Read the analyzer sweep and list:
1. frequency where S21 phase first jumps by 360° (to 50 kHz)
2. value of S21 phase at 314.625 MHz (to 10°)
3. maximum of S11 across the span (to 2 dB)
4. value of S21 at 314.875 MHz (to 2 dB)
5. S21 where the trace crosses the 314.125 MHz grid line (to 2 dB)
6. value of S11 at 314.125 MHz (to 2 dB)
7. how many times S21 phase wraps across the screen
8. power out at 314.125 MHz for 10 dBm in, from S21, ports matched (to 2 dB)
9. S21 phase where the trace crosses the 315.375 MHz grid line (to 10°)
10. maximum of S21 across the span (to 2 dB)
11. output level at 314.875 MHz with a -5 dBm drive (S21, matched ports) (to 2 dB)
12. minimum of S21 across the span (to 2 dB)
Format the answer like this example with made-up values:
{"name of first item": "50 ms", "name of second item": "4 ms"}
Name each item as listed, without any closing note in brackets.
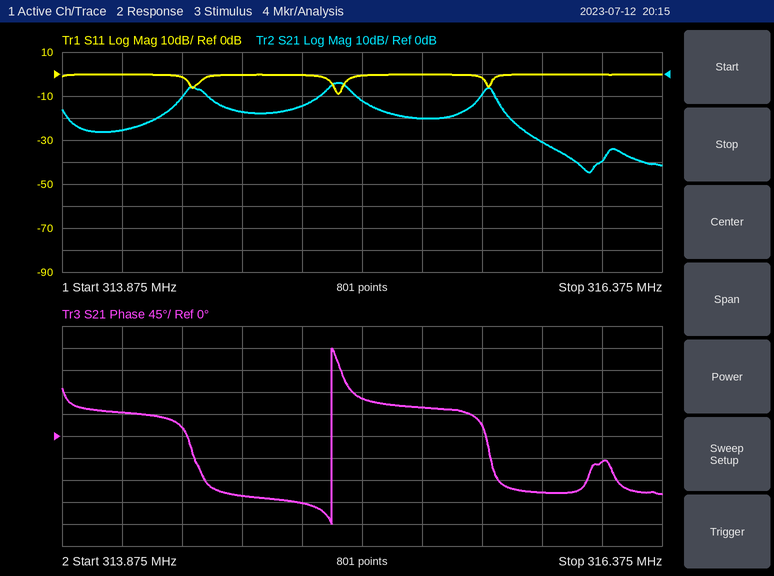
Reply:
{"frequency where S21 phase first jumps by 360°": "315.00 MHz", "value of S21 phase at 314.625 MHz": "-120°", "maximum of S11 across the span": "0 dB", "value of S21 at 314.875 MHz": "-14 dB", "S21 where the trace crosses the 314.125 MHz grid line": "-26 dB", "value of S11 at 314.125 MHz": "0 dB", "how many times S21 phase wraps across the screen": "1", "power out at 314.125 MHz for 10 dBm in, from S21, ports matched": "-16 dBm", "S21 phase where the trace crosses the 315.375 MHz grid line": "60°", "maximum of S21 across the span": "-4 dB", "output level at 314.875 MHz with a -5 dBm drive (S21, matched ports)": "-20 dBm", "minimum of S21 across the span": "-44 dB"}
